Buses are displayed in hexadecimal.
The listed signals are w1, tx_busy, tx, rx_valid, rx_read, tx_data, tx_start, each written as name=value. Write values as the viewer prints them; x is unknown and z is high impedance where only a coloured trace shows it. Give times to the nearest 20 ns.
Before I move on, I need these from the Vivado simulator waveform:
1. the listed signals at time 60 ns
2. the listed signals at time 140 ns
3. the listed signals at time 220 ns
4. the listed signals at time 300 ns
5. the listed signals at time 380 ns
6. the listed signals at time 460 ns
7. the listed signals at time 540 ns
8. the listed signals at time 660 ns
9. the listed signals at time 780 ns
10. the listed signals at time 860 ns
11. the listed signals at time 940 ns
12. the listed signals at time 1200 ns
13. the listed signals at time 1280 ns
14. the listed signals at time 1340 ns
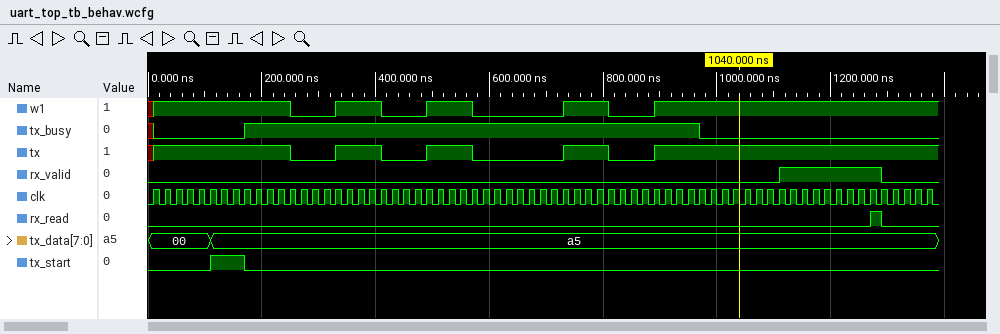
w1=1, tx_busy=0, tx=1, rx_valid=0, rx_read=0, tx_data=00, tx_start=0
w1=1, tx_busy=0, tx=1, rx_valid=0, rx_read=0, tx_data=a5, tx_start=1
w1=1, tx_busy=1, tx=1, rx_valid=0, rx_read=0, tx_data=a5, tx_start=0
w1=0, tx_busy=1, tx=0, rx_valid=0, rx_read=0, tx_data=a5, tx_start=0
w1=1, tx_busy=1, tx=1, rx_valid=0, rx_read=0, tx_data=a5, tx_start=0
w1=0, tx_busy=1, tx=0, rx_valid=0, rx_read=0, tx_data=a5, tx_start=0
w1=1, tx_busy=1, tx=1, rx_valid=0, rx_read=0, tx_data=a5, tx_start=0
w1=0, tx_busy=1, tx=0, rx_valid=0, rx_read=0, tx_data=a5, tx_start=0
w1=1, tx_busy=1, tx=1, rx_valid=0, rx_read=0, tx_data=a5, tx_start=0
w1=0, tx_busy=1, tx=0, rx_valid=0, rx_read=0, tx_data=a5, tx_start=0
w1=1, tx_busy=1, tx=1, rx_valid=0, rx_read=0, tx_data=a5, tx_start=0
w1=1, tx_busy=0, tx=1, rx_valid=1, rx_read=0, tx_data=a5, tx_start=0
w1=1, tx_busy=0, tx=1, rx_valid=1, rx_read=1, tx_data=a5, tx_start=0
w1=1, tx_busy=0, tx=1, rx_valid=0, rx_read=0, tx_data=a5, tx_start=0
